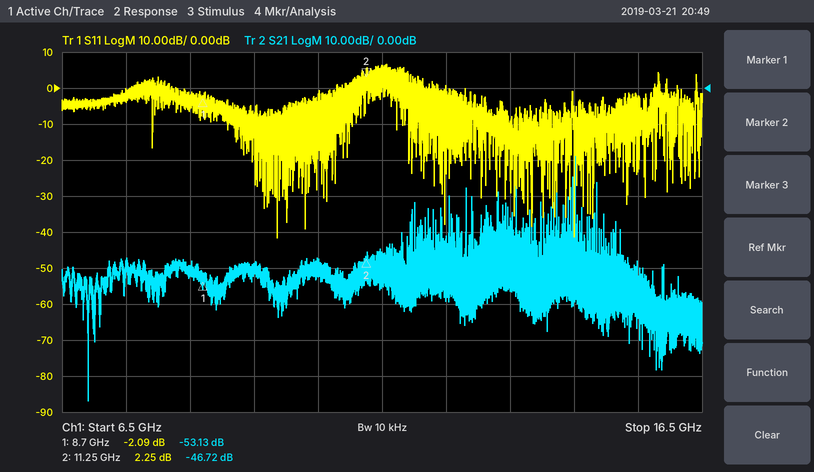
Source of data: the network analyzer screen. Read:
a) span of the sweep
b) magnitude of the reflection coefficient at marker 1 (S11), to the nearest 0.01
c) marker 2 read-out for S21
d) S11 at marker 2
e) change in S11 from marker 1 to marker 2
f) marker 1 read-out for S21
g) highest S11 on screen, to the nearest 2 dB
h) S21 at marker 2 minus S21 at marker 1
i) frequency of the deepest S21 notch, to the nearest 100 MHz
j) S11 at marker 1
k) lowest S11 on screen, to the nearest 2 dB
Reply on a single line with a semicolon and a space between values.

10 GHz; 0.79; -46.72 dB; 2.25 dB; 4.34 dB; -53.13 dB; 6 dB; 6.41 dB; 6.9 GHz; -2.09 dB; -42 dB
